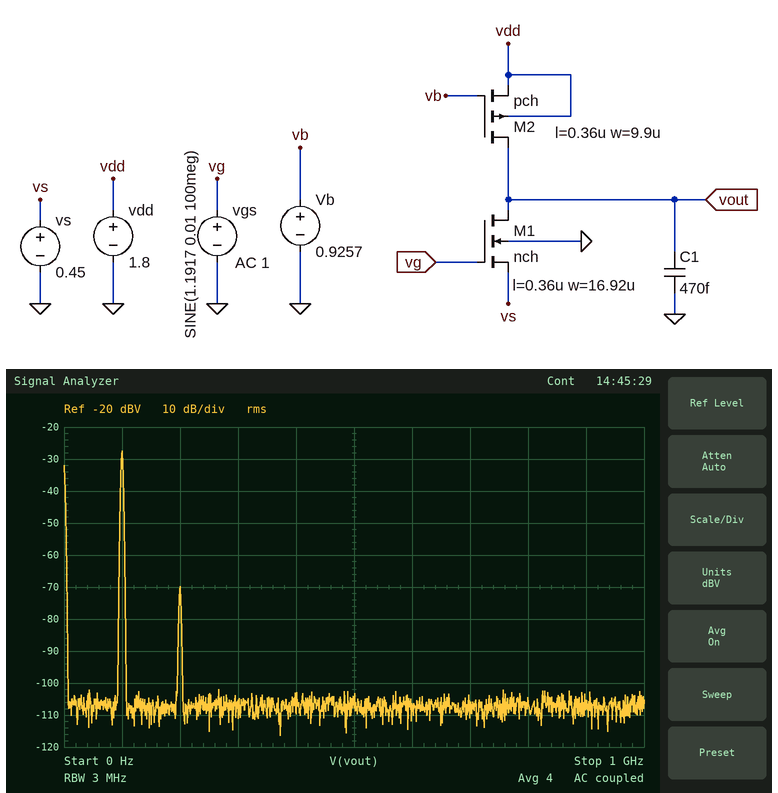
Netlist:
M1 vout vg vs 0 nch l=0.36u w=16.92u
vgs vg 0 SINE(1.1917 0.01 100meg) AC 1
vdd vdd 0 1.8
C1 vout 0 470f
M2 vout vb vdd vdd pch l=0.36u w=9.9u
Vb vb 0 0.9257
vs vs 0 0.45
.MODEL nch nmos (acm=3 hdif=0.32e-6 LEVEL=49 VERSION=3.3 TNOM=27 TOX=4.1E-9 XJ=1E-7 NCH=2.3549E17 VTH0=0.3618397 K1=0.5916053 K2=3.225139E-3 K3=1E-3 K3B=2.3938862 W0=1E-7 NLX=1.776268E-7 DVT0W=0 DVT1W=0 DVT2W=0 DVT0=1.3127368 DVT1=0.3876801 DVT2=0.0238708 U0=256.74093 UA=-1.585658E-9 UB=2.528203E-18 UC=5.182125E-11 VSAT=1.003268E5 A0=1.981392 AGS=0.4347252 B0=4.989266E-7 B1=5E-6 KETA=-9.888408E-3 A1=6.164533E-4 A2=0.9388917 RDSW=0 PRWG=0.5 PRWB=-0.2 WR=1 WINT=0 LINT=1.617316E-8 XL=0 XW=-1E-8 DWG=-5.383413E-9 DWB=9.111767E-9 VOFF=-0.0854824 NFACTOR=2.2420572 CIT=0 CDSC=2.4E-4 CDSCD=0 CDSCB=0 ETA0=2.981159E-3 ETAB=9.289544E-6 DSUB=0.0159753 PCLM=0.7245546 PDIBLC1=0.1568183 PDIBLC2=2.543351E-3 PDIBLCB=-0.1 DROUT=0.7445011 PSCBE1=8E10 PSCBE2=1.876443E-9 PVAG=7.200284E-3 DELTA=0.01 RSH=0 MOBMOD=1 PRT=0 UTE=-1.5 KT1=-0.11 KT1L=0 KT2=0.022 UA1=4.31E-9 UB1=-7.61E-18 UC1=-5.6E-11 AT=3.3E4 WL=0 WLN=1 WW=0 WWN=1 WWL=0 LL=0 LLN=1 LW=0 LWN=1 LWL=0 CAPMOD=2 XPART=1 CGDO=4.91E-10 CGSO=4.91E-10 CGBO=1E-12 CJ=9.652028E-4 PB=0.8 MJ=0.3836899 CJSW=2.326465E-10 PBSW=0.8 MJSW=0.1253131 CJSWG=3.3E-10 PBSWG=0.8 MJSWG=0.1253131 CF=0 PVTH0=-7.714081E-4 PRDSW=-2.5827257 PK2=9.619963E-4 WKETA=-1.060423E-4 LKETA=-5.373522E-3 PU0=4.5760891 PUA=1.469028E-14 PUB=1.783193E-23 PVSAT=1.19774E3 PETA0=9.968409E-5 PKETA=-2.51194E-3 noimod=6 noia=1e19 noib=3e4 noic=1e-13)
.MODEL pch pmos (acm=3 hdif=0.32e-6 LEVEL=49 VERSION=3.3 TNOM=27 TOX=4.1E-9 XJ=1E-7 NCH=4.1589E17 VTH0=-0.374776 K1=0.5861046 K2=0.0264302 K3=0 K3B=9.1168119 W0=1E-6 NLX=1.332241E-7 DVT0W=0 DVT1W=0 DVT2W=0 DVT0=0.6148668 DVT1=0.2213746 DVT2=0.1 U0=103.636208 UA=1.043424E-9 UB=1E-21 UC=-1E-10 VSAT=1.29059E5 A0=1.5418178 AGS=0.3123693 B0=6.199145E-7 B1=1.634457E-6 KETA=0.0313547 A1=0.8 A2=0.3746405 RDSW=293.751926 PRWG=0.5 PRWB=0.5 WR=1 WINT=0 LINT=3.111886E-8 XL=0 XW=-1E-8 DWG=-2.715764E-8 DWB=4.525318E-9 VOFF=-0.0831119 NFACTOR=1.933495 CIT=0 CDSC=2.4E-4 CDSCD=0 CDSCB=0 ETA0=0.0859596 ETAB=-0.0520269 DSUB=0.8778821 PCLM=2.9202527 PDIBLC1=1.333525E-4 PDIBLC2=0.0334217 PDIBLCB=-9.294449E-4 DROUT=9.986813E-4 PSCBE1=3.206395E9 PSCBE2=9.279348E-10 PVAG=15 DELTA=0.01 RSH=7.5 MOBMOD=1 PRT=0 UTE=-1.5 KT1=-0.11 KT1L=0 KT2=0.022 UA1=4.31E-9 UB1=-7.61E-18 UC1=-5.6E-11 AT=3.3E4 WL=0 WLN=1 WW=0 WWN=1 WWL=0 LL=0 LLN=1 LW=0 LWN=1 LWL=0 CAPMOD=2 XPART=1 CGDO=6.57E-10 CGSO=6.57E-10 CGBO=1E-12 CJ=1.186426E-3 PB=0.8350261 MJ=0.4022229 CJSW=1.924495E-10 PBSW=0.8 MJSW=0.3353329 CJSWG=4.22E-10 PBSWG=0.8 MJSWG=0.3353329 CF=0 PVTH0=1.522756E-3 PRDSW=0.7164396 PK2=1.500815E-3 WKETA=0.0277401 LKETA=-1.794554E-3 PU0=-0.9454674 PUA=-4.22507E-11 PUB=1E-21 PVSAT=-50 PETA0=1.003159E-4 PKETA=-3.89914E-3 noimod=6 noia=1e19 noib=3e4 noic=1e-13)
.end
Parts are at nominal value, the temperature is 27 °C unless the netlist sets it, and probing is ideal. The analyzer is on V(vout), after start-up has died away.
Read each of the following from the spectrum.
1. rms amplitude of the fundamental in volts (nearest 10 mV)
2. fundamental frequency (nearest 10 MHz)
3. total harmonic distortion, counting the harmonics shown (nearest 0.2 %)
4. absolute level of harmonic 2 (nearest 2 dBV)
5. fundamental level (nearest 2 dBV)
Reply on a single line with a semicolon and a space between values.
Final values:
40 mV; 100 MHz; 0.8 %; -70 dBV; -28 dBV
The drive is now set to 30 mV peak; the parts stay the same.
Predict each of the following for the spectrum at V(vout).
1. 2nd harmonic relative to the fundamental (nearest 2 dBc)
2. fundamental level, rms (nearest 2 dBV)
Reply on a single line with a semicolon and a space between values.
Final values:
-32 dBc; -18 dBV
